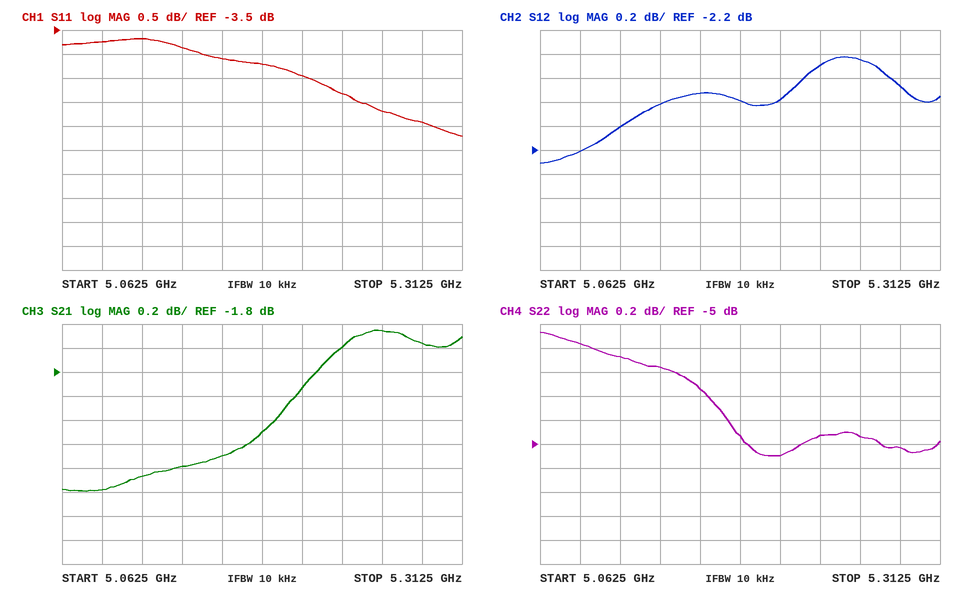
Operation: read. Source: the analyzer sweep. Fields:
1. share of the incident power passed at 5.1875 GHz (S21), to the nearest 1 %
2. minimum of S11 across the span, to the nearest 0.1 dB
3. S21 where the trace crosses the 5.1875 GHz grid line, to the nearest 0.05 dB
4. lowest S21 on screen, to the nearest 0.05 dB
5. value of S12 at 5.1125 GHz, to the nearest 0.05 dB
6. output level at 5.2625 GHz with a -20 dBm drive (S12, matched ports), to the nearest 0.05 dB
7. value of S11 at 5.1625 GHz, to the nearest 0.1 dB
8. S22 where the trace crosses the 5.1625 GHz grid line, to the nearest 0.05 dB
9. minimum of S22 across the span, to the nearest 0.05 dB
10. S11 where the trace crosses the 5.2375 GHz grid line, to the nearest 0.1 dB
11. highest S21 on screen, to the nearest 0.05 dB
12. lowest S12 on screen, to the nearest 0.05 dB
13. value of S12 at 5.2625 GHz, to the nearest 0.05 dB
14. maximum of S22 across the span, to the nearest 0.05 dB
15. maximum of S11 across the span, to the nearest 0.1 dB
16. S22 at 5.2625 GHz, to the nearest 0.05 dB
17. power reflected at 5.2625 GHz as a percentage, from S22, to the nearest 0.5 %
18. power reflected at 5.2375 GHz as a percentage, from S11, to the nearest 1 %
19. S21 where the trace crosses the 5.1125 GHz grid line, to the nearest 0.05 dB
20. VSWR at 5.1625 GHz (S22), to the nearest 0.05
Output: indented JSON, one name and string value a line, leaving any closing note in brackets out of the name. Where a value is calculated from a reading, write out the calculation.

{
  "share of the incident power passed at 5.1875 GHz (S21), to the nearest 1 %": "10^(-2.3/10) ≈ 59 %",
  "minimum of S11 across the span, to the nearest 0.1 dB": "-5.7 dB",
  "S21 where the trace crosses the 5.1875 GHz grid line, to the nearest 0.05 dB": "-2.30 dB",
  "lowest S21 on screen, to the nearest 0.05 dB": "-2.80 dB",
  "value of S12 at 5.1125 GHz, to the nearest 0.05 dB": "-2.00 dB",
  "output level at 5.2625 GHz with a -20 dBm drive (S12, matched ports), to the nearest 0.05 dB": "-20 dBm + (-1.45 dB) = -21.45 dBm",
  "value of S11 at 5.1625 GHz, to the nearest 0.1 dB": "-4.1 dB",
  "S22 where the trace crosses the 5.1625 GHz grid line, to the nearest 0.05 dB": "-4.55 dB",
  "minimum of S22 across the span, to the nearest 0.05 dB": "-5.10 dB",
  "S11 where the trace crosses the 5.2375 GHz grid line, to the nearest 0.1 dB": "-4.8 dB",
  "highest S21 on screen, to the nearest 0.05 dB": "-1.45 dB",
  "lowest S12 on screen, to the nearest 0.05 dB": "-2.30 dB",
  "value of S12 at 5.2625 GHz, to the nearest 0.05 dB": "-1.45 dB",
  "maximum of S22 across the span, to the nearest 0.05 dB": "-4.05 dB",
  "maximum of S11 across the span, to the nearest 0.1 dB": "-3.7 dB",
  "S22 at 5.2625 GHz, to the nearest 0.05 dB": "-4.95 dB",
  "power reflected at 5.2625 GHz as a percentage, from S22, to the nearest 0.5 %": "10^(-4.95/10) ≈ 32.0 %",
  "power reflected at 5.2375 GHz as a percentage, from S11, to the nearest 1 %": "10^(-4.8/10) ≈ 33 %",
  "S21 where the trace crosses the 5.1125 GHz grid line, to the nearest 0.05 dB": "-2.65 dB",
  "VSWR at 5.1625 GHz (S22), to the nearest 0.05": "|Γ| = 10^(-4.55/20) = 0.5922; VSWR = (1 + 0.5922)/(1 − 0.5922) ≈ 3.90"
}
